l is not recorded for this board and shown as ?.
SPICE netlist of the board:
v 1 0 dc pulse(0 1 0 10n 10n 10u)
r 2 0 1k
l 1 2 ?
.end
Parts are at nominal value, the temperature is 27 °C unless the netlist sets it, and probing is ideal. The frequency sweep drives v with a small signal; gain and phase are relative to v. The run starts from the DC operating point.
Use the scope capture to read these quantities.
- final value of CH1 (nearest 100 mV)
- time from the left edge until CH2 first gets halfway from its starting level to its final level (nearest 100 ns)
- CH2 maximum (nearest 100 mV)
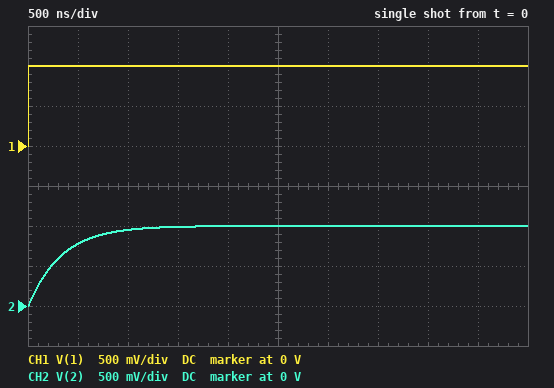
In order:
1.0 V
200 ns
1.0 V
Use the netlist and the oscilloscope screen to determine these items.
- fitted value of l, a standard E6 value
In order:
330 µH
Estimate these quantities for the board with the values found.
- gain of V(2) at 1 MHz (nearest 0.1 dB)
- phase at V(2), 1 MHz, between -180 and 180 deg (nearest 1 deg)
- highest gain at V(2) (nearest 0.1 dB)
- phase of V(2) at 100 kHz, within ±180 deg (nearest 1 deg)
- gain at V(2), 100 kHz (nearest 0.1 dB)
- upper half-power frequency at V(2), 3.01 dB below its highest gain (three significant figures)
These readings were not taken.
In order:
-7.2 dB
-64 deg
0 dB
-12 deg
-0.2 dB
482 kHz
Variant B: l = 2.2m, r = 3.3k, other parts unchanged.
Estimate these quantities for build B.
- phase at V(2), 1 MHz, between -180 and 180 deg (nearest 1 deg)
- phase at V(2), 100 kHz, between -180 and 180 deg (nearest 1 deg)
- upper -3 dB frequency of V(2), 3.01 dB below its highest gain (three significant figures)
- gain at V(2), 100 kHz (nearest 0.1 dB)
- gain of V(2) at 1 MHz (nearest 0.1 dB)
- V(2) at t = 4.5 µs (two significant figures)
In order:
-77 deg
-23 deg
239 kHz
-0.7 dB
-12.7 dB
1.0 V
